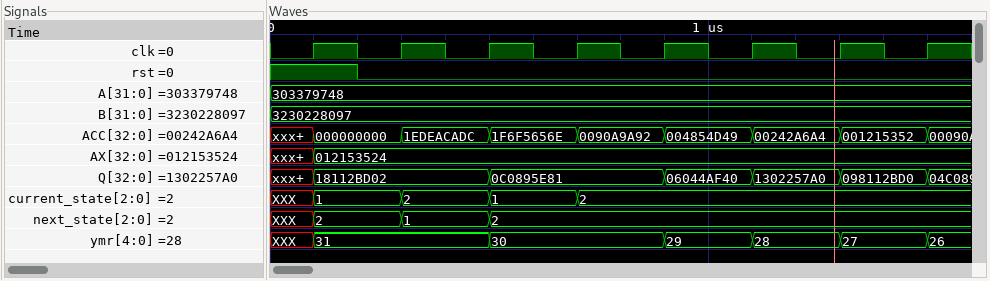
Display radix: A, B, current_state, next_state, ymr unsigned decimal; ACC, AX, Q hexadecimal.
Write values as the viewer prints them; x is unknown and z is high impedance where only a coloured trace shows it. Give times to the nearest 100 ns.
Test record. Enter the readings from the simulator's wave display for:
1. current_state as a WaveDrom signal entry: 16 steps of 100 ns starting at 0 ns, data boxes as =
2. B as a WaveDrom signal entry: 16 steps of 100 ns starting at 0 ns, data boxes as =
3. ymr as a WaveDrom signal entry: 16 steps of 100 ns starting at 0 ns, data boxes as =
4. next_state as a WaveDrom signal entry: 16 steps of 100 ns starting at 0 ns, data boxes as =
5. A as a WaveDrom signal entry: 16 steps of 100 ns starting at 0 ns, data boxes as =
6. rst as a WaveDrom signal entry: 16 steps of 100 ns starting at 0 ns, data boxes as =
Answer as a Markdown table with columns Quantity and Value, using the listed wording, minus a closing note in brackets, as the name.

| Quantity | Value |
|---|---|
| current_state as a WaveDrom signal entry: 16 steps of 100 ns starting at 0 ns, data boxes as = | {name: 'current_state', wave: 'x=.=.=.=........', data: '1 2 1 2'} |
| B as a WaveDrom signal entry: 16 steps of 100 ns starting at 0 ns, data boxes as = | {name: 'B', wave: '=...............', data: '3230228097'} |
| ymr as a WaveDrom signal entry: 16 steps of 100 ns starting at 0 ns, data boxes as = | {name: 'ymr', wave: 'x=...=...=.=.=.=', data: '31 30 29 28 27 26'} |
| next_state as a WaveDrom signal entry: 16 steps of 100 ns starting at 0 ns, data boxes as = | {name: 'next_state', wave: 'x=.=.=..........', data: '2 1 2'} |
| A as a WaveDrom signal entry: 16 steps of 100 ns starting at 0 ns, data boxes as = | {name: 'A', wave: '=...............', data: '303379748'} |
| rst as a WaveDrom signal entry: 16 steps of 100 ns starting at 0 ns, data boxes as = | {name: 'rst', wave: '1.0.............'} |
